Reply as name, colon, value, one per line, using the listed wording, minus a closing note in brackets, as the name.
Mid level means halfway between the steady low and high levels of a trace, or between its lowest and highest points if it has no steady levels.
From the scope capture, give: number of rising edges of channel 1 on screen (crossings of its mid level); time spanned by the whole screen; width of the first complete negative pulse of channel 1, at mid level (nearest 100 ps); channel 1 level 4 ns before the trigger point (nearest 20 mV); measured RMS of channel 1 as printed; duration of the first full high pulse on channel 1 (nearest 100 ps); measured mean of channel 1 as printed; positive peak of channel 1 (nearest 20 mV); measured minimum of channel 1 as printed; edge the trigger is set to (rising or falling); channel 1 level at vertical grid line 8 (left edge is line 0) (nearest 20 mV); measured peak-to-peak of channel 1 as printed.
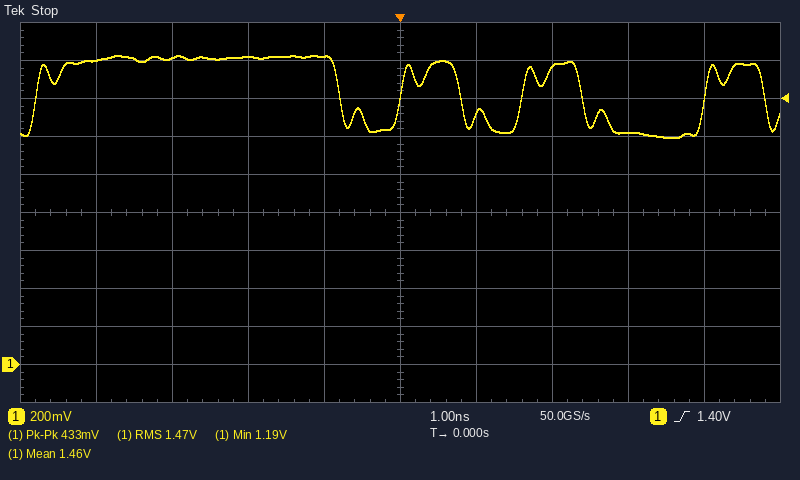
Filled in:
number of rising edges of channel 1 on screen: 4
time spanned by the whole screen: 10 ns
width of the first complete negative pulse of channel 1, at mid level: 800 ps
channel 1 level 4 ns before the trigger point: 1.60 V
measured RMS of channel 1 as printed: 1.47 V
duration of the first full high pulse on channel 1: 4.0 ns
measured mean of channel 1 as printed: 1.46 V
positive peak of channel 1: 1.62 V
measured minimum of channel 1 as printed: 1.19 V
edge the trigger is set to: rising
channel 1 level at vertical grid line 8 (left edge is line 0): 1.22 V
measured peak-to-peak of channel 1 as printed: 433 mV
